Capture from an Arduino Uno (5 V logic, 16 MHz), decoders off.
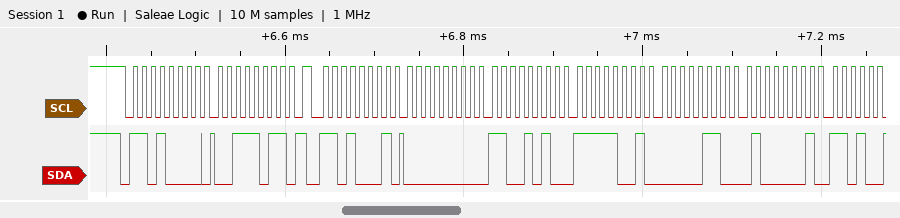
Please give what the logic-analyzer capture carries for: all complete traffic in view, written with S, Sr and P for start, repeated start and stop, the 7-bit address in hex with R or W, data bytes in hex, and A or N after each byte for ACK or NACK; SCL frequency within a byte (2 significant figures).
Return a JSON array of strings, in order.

["S 68W A 3B A Sr 68R A 00 A CA A F9 A 06 A 41 A", "100 kHz"]
